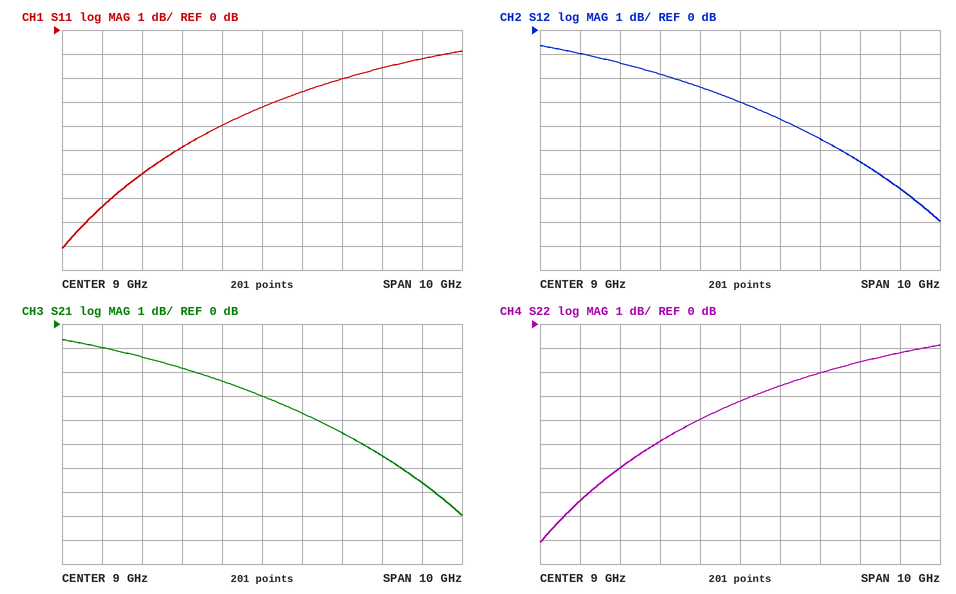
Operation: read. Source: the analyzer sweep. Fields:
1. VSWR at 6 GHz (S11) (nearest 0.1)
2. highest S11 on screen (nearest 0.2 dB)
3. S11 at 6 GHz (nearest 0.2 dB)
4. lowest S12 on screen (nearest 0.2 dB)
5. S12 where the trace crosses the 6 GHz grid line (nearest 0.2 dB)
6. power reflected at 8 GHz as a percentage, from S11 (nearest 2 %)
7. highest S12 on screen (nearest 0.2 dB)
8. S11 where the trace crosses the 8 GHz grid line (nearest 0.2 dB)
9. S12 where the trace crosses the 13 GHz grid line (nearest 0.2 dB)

3.0
-0.8 dB
-6.0 dB
-8.0 dB
-1.4 dB
40 %
-0.6 dB
-4.0 dB
-6.6 dB
